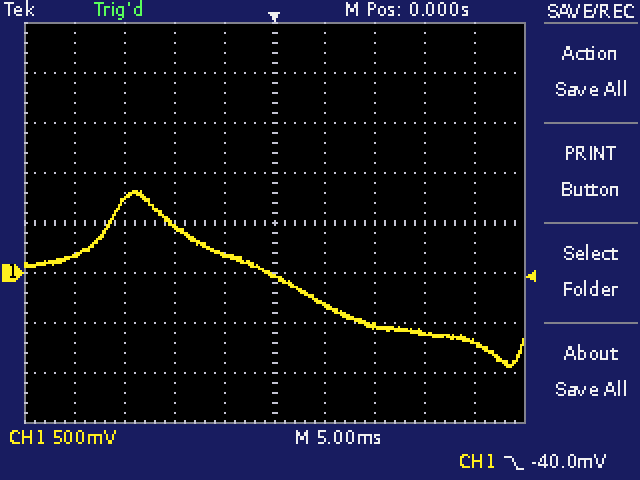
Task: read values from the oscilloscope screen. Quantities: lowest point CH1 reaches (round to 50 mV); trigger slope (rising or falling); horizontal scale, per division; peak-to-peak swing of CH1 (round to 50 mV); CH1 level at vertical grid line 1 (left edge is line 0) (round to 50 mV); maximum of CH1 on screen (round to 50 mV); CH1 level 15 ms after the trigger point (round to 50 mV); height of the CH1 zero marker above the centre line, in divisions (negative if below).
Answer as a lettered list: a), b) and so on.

a) -950 mV
b) falling
c) 5 ms
d) 1.75 V
e) 200 mV
f) 800 mV
g) -600 mV
h) -1.0 div
